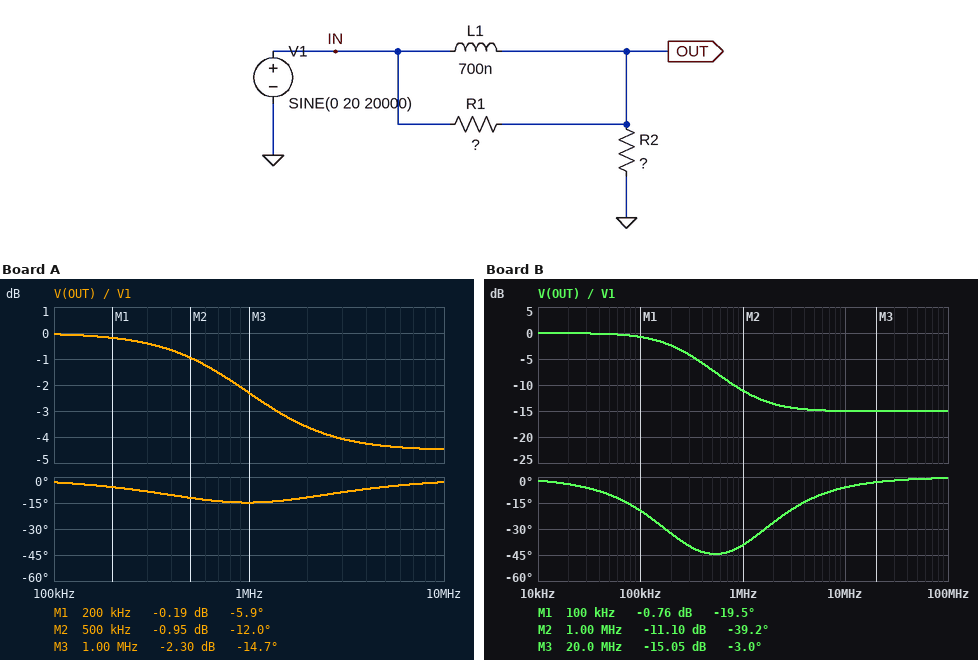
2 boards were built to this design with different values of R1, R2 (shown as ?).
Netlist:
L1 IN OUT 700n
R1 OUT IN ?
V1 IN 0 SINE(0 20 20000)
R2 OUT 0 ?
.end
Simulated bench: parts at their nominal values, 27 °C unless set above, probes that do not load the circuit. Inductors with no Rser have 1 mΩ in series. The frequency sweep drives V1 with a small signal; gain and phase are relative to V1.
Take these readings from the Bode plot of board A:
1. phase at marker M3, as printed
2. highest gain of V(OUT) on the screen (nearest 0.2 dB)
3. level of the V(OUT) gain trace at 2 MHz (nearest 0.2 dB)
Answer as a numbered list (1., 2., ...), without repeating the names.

1. -14.7 deg
2. 0 dB
3. -3.6 dB
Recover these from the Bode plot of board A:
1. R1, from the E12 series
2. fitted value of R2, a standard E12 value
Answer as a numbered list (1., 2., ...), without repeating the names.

1. 5.6 Ω
2. 8.2 Ω
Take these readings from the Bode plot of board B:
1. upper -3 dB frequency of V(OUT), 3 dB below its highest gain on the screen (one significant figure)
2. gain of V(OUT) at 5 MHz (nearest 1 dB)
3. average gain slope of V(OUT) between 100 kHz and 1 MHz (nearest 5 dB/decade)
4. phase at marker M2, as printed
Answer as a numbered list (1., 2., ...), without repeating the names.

1. 200 kHz
2. -15 dB
3. -10 dB/decade
4. -39.2 deg
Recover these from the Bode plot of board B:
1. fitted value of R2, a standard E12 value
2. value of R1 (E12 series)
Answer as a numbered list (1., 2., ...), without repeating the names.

1. 1.2 Ω
2. 5.6 Ω
